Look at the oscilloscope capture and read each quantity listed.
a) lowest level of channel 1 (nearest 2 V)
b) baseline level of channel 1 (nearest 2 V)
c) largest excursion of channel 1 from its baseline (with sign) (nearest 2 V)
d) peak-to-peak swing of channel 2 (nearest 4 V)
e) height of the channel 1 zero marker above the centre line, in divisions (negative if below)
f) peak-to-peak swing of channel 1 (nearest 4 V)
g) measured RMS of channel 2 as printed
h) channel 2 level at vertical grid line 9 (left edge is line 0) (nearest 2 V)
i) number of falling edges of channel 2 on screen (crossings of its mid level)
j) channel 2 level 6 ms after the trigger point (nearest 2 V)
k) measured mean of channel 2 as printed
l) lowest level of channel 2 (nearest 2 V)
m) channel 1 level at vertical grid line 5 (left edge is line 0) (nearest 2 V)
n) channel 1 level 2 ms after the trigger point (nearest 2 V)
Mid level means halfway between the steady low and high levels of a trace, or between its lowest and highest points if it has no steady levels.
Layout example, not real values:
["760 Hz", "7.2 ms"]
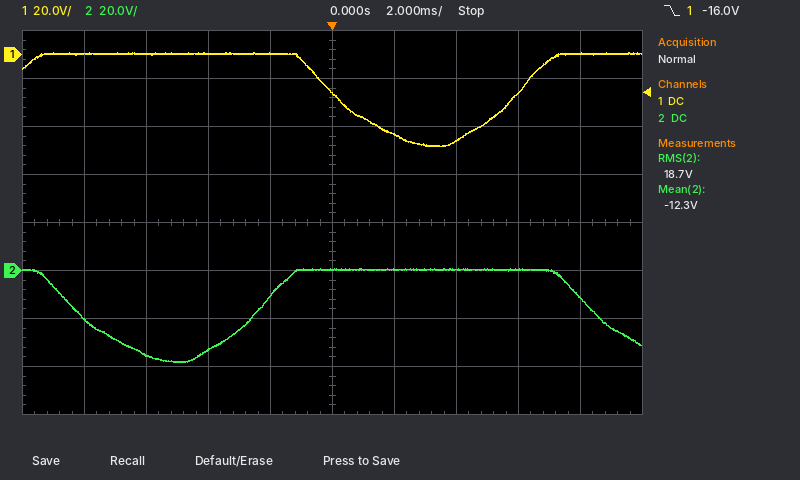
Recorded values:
["-38 V", "0 V", "-38 V", "40 V", "+3.5 div", "40 V", "18.7 V", "-12 V", "2", "0 V", "-12.3 V", "-38 V", "-16 V", "-34 V"]
